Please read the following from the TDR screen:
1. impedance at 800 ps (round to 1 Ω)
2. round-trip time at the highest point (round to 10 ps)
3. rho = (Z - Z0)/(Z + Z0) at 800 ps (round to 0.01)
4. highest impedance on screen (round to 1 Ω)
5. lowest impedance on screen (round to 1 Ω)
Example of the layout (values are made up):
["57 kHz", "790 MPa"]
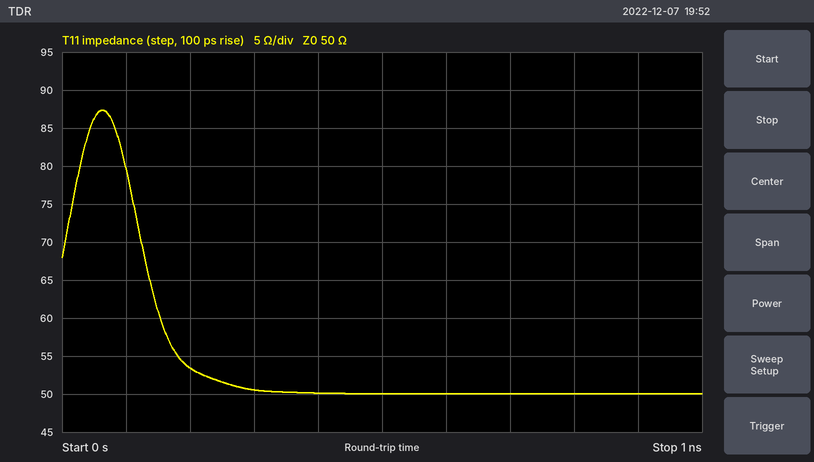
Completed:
["50 Ω", "60 ps", "0.00", "87 Ω", "50 Ω"]
